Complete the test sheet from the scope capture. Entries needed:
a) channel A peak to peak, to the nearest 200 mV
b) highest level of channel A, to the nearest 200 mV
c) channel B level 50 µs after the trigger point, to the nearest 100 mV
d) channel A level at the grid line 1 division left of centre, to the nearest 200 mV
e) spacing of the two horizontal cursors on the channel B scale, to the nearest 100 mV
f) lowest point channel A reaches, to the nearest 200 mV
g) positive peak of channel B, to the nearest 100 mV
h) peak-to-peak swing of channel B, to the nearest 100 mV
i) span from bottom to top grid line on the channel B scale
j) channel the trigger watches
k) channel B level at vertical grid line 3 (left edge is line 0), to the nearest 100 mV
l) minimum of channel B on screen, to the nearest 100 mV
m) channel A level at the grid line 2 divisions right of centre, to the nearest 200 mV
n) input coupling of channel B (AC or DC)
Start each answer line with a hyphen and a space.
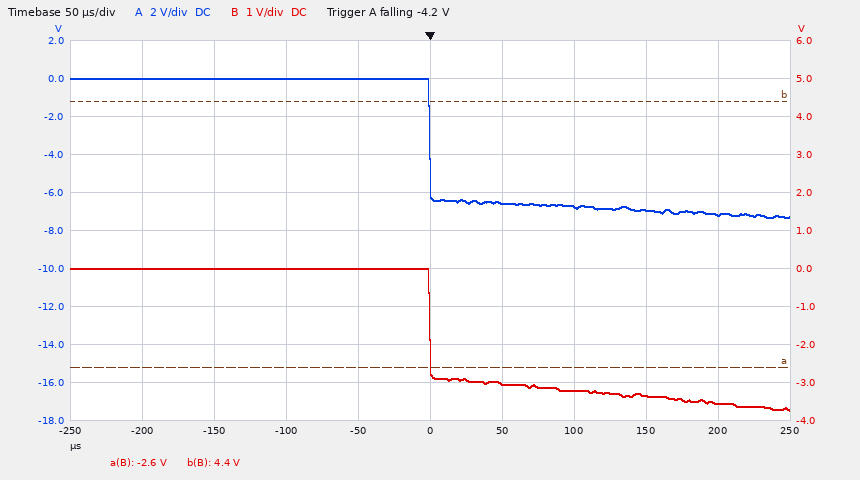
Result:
- 7.4 V
- 0.0 V
- -3.0 V
- 0.0 V
- 7.0 V
- -7.4 V
- 0.0 V
- 3.7 V
- 10 V
- channel A
- 0.0 V
- -3.7 V
- -6.8 V
- DC
